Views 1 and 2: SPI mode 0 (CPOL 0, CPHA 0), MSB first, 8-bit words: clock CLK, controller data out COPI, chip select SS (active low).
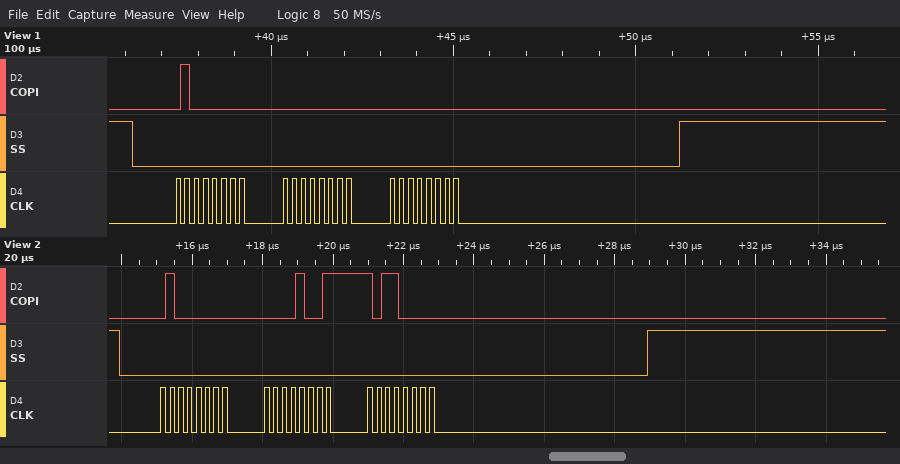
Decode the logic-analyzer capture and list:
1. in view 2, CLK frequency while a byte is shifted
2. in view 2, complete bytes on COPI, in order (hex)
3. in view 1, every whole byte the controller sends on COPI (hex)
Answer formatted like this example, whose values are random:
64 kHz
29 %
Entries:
4 MHz
0x40 0x09 0xB0
40 00 00
